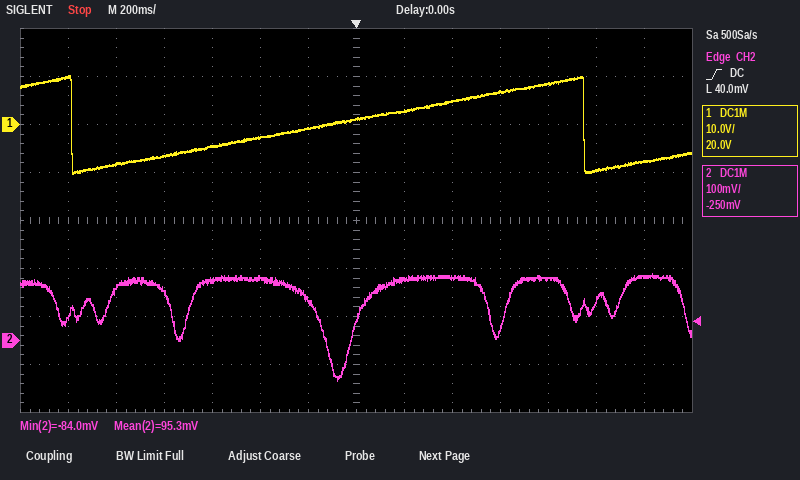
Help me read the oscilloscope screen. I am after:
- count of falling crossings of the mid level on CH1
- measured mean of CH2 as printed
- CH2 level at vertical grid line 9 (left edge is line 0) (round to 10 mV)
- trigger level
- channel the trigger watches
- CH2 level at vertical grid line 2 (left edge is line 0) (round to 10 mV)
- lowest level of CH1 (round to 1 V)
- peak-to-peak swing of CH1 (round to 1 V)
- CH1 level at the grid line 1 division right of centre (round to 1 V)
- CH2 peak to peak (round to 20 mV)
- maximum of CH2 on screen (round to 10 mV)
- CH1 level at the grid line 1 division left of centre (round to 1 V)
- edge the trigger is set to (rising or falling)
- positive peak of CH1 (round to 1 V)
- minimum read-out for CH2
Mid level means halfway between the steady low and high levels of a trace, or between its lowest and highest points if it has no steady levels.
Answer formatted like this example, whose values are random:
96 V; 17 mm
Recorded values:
2; 95.3 mV; 130 mV; 40.0 mV; CH2; 110 mV; -10 V; 20 V; 3 V; 220 mV; 140 mV; -1 V; rising; 10 V; -84.0 mV
